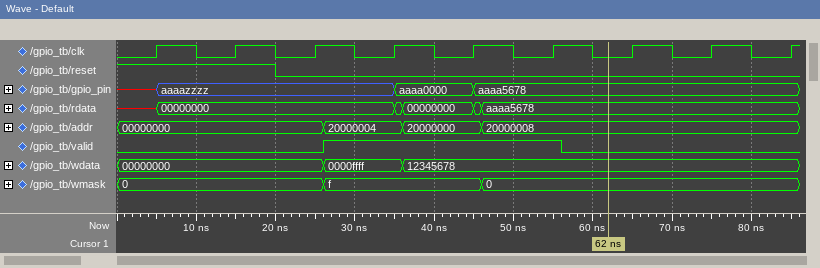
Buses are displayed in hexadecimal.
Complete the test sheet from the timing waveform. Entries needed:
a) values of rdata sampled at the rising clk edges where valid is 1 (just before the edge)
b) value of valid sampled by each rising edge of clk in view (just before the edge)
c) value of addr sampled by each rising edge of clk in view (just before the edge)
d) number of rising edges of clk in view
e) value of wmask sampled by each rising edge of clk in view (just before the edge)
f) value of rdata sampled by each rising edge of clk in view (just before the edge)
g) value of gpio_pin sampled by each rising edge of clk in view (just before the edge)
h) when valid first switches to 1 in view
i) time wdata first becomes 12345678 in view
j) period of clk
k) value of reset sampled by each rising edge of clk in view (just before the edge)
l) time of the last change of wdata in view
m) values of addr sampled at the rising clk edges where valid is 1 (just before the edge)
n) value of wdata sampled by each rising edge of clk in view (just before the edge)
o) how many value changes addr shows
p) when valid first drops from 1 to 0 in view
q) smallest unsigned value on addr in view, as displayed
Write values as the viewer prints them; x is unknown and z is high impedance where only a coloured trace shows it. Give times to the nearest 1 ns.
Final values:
00000000, 00000000, aaaa5678
0 0 0 1 1 1 0 0 0
00000000, 00000000, 00000000, 20000004, 20000000, 20000008, 20000008, 20000008, 20000008
9
0, 0, 0, f, f, 0, 0, 0, 0
x, 00000000, 00000000, 00000000, 00000000, aaaa5678, aaaa5678, aaaa5678, aaaa5678
x, aaaazzzz, aaaazzzz, aaaazzzz, aaaa0000, aaaa5678, aaaa5678, aaaa5678, aaaa5678
26 ns
36 ns
10 ns
1 1 0 0 0 0 0 0 0
36 ns
20000004, 20000000, 20000008
00000000, 00000000, 00000000, 0000ffff, 12345678, 12345678, 12345678, 12345678, 12345678
3
56 ns
00000000
